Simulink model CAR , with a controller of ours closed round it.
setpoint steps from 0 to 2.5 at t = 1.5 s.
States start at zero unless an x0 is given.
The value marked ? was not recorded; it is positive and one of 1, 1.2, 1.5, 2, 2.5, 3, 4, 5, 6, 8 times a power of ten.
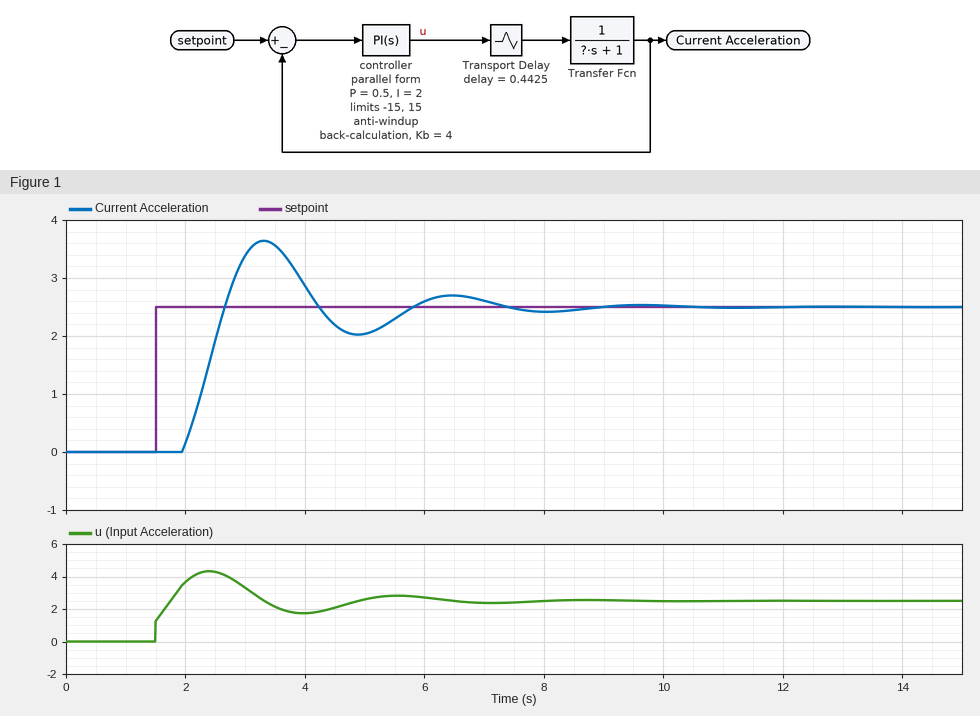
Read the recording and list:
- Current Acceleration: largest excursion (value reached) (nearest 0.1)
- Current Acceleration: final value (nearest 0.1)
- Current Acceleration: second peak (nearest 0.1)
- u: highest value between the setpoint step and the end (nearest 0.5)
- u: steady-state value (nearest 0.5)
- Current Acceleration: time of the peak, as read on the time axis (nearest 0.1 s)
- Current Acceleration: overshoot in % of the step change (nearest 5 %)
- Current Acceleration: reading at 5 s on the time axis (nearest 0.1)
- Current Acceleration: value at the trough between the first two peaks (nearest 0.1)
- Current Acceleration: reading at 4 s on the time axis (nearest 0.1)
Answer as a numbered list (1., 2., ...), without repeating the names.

1. 3.6
2. 2.5
3. 2.7
4. 4.5
5. 2.5
6. 3.3 s
7. 45 %
8. 2.0
9. 2.0
10. 2.9
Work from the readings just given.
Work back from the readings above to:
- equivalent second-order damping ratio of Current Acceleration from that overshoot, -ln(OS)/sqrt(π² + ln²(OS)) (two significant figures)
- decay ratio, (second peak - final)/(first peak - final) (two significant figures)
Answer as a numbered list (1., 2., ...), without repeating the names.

1. 0.25
2. 0.18
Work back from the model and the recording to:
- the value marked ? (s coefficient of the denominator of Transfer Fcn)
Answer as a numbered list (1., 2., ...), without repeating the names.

1. 0.5
